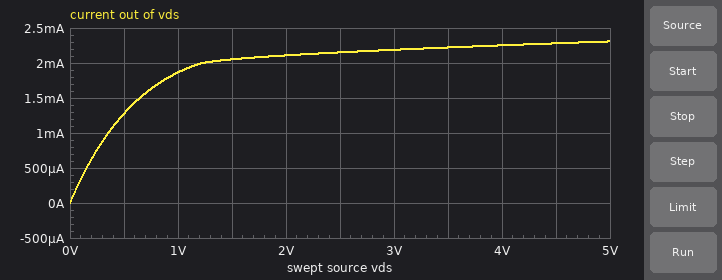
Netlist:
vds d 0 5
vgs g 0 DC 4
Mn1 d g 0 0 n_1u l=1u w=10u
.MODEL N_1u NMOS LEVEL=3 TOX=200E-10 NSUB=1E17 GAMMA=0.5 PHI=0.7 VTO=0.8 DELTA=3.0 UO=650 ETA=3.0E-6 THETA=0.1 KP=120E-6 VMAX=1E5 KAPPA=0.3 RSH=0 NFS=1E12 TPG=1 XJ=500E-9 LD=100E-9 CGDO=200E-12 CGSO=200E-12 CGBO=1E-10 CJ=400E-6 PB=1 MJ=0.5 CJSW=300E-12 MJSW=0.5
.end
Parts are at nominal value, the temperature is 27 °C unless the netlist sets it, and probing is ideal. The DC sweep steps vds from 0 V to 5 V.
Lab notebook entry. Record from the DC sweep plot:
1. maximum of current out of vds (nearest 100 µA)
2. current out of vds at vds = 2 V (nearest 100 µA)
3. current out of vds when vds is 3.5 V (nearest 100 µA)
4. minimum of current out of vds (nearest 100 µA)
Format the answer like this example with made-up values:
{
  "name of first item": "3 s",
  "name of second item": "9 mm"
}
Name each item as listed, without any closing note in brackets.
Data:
{
  "maximum of current out of vds": "2.3 mA",
  "current out of vds at vds = 2 V": "2.1 mA",
  "current out of vds when vds is 3.5 V": "2.2 mA",
  "minimum of current out of vds": "0 A"
}
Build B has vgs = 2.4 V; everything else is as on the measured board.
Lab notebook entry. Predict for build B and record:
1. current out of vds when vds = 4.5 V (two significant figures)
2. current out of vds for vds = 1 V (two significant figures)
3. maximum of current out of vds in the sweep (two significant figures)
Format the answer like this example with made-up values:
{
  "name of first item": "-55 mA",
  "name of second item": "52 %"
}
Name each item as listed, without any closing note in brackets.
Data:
{
  "current out of vds when vds = 4.5 V": "910 µA",
  "current out of vds for vds = 1 V": "800 µA",
  "maximum of current out of vds in the sweep": "920 µA"
}
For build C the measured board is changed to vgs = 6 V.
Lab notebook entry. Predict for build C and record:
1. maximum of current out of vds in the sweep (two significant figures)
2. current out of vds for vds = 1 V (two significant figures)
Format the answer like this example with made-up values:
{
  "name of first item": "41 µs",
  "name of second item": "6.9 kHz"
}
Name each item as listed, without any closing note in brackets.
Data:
{
  "maximum of current out of vds in the sweep": "4.1 mA",
  "current out of vds for vds = 1 V": "3.0 mA"
}
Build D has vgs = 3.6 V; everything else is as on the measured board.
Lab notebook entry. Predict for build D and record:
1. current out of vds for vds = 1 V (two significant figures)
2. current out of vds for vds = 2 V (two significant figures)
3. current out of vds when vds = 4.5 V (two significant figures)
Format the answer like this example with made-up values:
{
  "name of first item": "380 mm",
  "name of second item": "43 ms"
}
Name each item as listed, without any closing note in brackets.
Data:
{
  "current out of vds for vds = 1 V": "1.6 mA",
  "current out of vds for vds = 2 V": "1.8 mA",
  "current out of vds when vds = 4.5 V": "1.9 mA"
}
